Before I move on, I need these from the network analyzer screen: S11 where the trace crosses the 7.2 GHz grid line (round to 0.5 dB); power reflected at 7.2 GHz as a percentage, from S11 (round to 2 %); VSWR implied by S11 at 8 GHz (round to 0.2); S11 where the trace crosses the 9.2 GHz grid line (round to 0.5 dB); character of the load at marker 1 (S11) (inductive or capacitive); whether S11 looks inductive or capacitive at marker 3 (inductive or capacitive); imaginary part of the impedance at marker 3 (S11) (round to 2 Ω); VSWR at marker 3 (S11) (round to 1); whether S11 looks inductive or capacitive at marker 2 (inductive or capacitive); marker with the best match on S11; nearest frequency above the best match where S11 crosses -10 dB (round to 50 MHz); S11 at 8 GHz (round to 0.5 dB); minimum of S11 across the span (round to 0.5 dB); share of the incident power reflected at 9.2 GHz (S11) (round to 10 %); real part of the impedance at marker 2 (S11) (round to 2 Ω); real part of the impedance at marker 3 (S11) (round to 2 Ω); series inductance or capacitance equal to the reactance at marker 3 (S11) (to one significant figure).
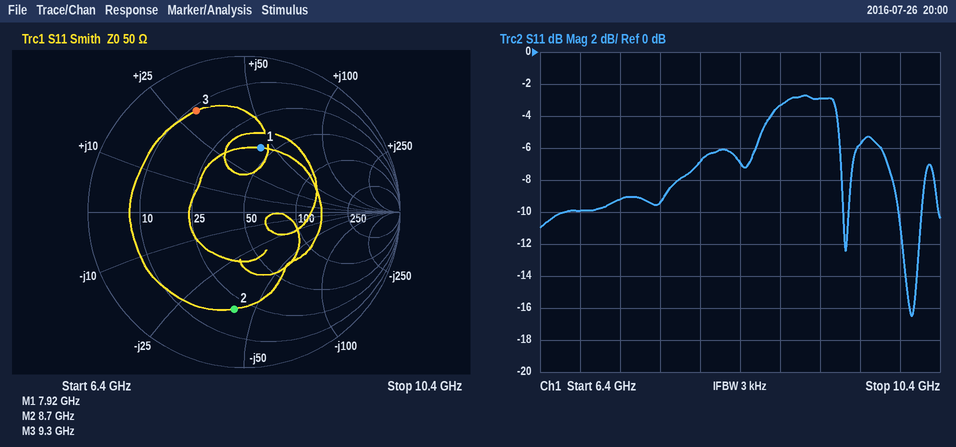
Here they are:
-9.0 dB
12 %
2.6
-3.0 dB
inductive
inductive
+30 Ω
6
capacitive
marker 1
10.20 GHz
-7.0 dB
-16.5 dB
50 %
20 Ω
12 Ω
500 pH
